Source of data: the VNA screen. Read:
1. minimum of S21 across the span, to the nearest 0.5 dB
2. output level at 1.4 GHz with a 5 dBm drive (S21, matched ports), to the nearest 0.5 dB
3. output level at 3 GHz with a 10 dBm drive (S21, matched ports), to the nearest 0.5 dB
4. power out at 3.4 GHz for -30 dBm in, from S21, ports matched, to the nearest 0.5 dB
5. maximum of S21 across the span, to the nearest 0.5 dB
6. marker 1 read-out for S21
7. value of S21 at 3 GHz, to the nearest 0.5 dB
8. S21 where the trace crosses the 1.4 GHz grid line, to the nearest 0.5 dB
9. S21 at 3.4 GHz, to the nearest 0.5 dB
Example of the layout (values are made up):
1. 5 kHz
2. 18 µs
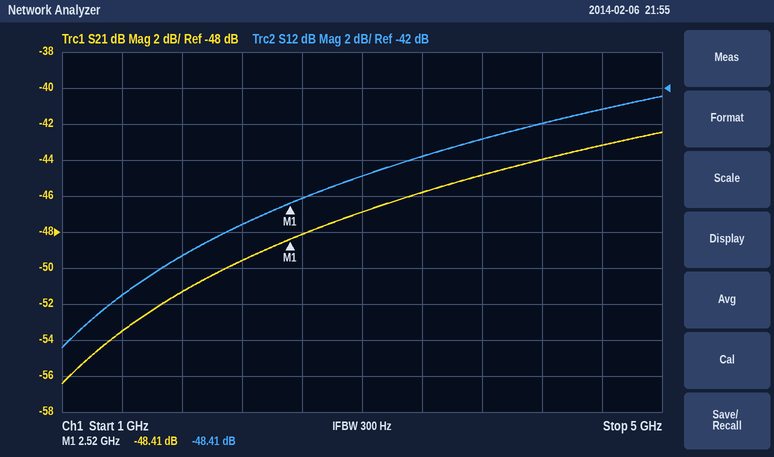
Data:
1. -56.5 dB
2. -48.5 dBm
3. -37.0 dBm
4. -76.0 dBm
5. -42.5 dB
6. -48.41 dB
7. -47.0 dB
8. -53.5 dB
9. -46.0 dB
